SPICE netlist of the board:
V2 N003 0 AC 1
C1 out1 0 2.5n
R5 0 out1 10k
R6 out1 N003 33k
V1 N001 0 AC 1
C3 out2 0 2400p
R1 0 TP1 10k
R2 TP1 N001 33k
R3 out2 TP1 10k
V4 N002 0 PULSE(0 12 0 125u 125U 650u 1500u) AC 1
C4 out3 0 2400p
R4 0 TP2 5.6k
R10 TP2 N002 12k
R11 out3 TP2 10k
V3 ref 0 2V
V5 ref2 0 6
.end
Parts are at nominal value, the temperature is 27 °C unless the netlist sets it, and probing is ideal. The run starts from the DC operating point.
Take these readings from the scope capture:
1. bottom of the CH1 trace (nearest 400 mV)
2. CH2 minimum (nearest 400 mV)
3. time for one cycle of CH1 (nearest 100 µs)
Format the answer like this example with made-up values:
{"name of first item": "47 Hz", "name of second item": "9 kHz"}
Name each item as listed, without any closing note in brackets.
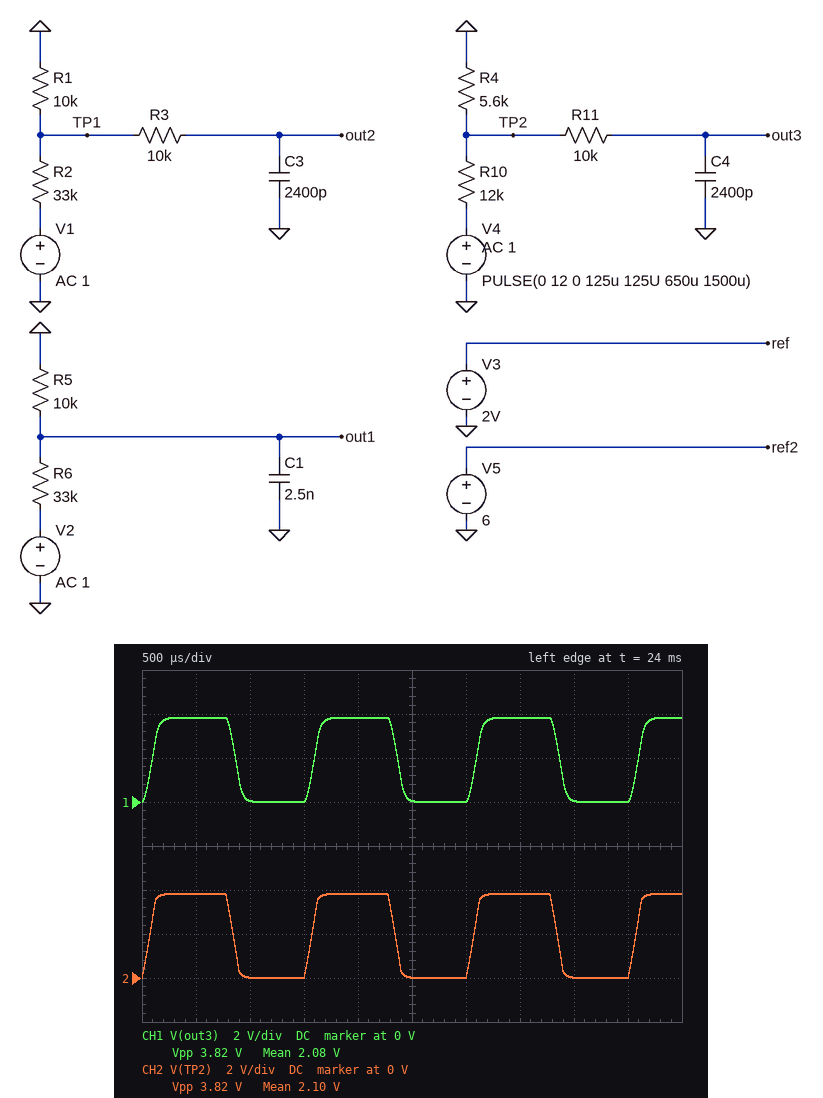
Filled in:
{"bottom of the CH1 trace": "0 V", "CH2 minimum": "0 V", "time for one cycle of CH1": "1.5 ms"}
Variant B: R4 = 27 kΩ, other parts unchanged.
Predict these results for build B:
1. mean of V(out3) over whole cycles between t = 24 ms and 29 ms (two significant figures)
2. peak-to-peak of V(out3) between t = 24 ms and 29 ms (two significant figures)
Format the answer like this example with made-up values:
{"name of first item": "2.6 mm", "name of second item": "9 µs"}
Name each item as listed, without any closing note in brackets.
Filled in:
{"mean of V(out3) over whole cycles between t = 24 ms and 29 ms": "4.3 V", "peak-to-peak of V(out3) between t = 24 ms and 29 ms": "8.3 V"}
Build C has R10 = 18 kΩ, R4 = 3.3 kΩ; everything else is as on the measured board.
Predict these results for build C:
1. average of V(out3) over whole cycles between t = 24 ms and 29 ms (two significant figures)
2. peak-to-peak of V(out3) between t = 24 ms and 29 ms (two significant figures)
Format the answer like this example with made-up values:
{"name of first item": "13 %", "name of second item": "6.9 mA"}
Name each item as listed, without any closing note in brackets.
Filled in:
{"average of V(out3) over whole cycles between t = 24 ms and 29 ms": "960 mV", "peak-to-peak of V(out3) between t = 24 ms and 29 ms": "1.9 V"}
